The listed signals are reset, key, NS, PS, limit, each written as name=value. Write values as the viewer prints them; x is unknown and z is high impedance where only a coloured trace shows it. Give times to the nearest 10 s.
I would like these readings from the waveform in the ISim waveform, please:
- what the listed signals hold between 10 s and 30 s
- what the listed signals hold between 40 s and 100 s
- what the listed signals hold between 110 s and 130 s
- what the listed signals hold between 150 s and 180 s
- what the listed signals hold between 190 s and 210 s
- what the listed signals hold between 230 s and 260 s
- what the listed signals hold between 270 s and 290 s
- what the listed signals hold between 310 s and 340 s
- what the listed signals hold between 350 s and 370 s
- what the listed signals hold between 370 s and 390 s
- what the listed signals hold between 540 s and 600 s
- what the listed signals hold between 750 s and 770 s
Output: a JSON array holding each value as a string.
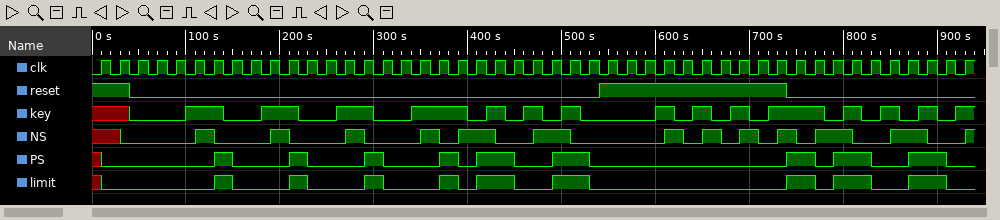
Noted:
["reset=1, key=x, NS=x, PS=0, limit=0", "reset=0, key=0, NS=0, PS=0, limit=0", "reset=0, key=1, NS=1, PS=0, limit=0", "reset=0, key=0, NS=0, PS=0, limit=0", "reset=0, key=1, NS=1, PS=0, limit=0", "reset=0, key=0, NS=0, PS=0, limit=0", "reset=0, key=1, NS=1, PS=0, limit=0", "reset=0, key=0, NS=0, PS=0, limit=0", "reset=0, key=1, NS=1, PS=0, limit=0", "reset=0, key=1, NS=0, PS=1, limit=1", "reset=1, key=0, NS=0, PS=0, limit=0", "reset=0, key=1, NS=0, PS=1, limit=1"]
